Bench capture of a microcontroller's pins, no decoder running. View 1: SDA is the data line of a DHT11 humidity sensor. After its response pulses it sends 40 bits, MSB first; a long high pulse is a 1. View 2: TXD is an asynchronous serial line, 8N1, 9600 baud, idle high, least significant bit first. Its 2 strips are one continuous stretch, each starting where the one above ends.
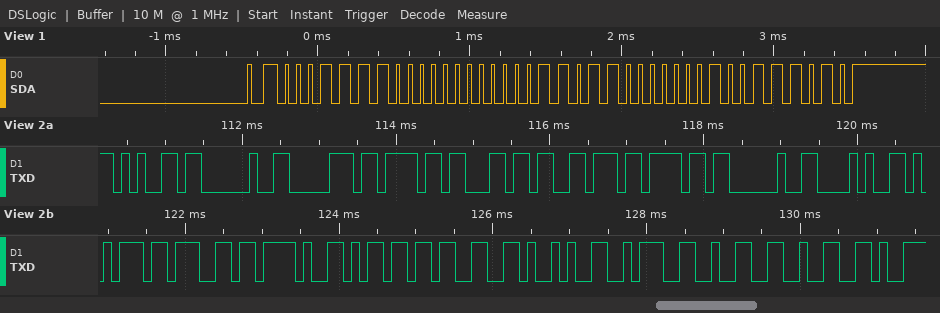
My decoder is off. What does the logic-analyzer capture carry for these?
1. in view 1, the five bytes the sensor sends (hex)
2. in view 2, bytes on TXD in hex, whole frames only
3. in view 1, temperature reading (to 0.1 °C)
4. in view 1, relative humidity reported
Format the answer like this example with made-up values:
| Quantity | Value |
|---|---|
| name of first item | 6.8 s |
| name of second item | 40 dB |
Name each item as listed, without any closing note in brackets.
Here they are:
| Quantity | Value |
|---|---|
| in view 1, the five bytes the sensor sends | 1E 00 1B 01 3A |
| in view 2, bytes on TXD in hex, whole frames only | 65 20 70 6F 6C 76 6F 20 28 75 67 2F 6D 33 29 3A 32 32 |
| in view 1, temperature reading | 27.1 °C |
| in view 1, relative humidity reported | 30 % |
